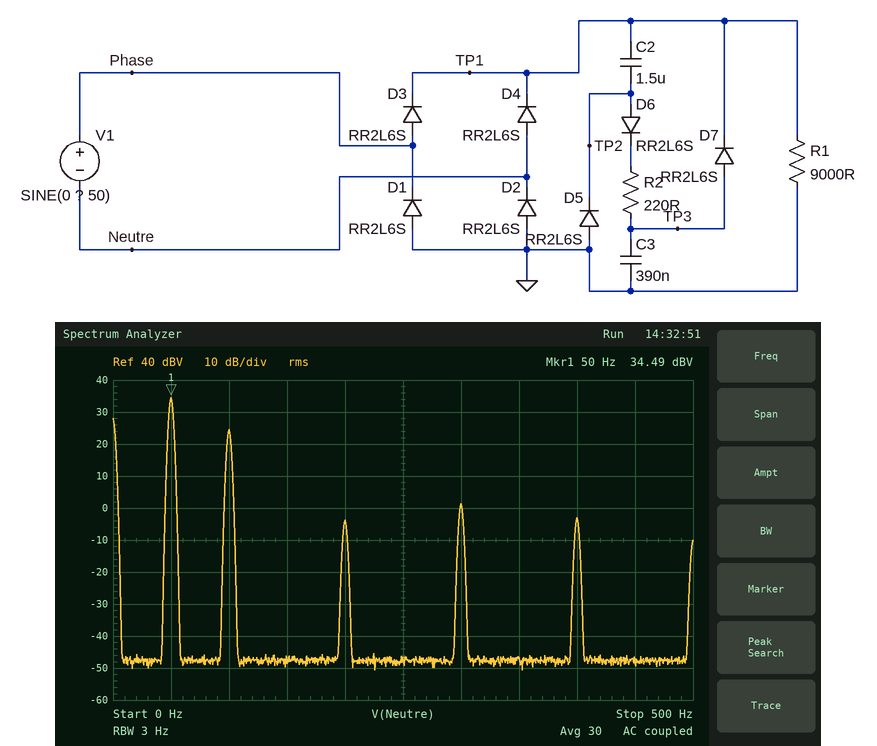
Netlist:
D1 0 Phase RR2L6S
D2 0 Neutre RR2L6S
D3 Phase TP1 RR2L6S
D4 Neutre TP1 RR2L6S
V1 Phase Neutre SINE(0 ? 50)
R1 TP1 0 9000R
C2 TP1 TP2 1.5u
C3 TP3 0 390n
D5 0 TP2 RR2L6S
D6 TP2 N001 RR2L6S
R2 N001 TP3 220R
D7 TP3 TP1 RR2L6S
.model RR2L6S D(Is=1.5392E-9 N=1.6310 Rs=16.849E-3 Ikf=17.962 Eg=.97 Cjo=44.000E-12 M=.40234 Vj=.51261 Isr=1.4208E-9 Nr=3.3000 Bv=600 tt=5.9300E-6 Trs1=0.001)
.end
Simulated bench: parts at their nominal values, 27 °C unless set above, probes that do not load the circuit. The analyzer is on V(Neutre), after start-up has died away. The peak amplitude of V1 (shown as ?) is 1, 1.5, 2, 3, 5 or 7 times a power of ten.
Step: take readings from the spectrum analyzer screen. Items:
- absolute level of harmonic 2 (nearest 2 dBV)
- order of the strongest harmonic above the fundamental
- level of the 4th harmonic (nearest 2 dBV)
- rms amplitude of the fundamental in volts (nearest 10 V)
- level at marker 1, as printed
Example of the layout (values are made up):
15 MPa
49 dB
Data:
24 dBV
2
-4 dBV
50 V
34.49 dBV
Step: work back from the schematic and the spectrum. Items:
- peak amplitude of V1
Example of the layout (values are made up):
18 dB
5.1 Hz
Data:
150 V
